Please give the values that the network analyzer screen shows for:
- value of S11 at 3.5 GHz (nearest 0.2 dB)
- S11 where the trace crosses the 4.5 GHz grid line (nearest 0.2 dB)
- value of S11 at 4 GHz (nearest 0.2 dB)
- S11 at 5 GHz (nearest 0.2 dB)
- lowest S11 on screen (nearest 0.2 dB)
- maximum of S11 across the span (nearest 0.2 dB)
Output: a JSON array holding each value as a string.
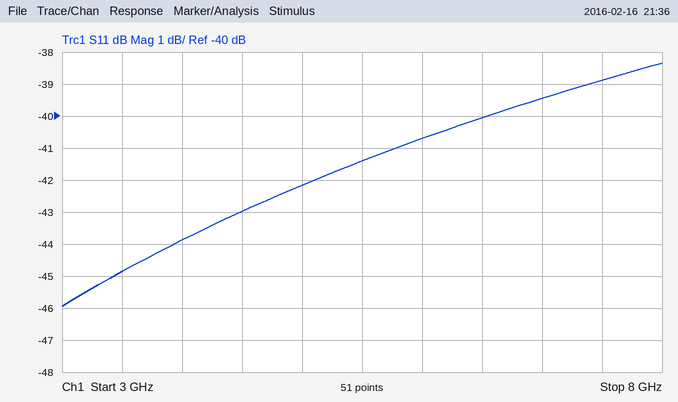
["-44.8 dB", "-43.0 dB", "-43.8 dB", "-42.2 dB", "-46.0 dB", "-38.4 dB"]
